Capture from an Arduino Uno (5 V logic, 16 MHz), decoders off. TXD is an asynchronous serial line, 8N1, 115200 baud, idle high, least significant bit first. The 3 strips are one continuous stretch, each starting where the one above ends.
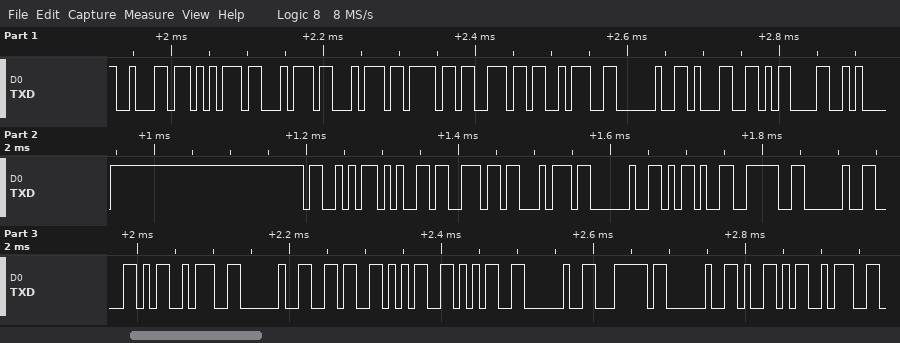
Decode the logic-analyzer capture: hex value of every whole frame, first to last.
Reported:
0x62 0x75 0x74 0x74 0x6F 0x6E 0x3A 0x20 0x31 0x0D 0x0A 0x53 0x65 0x6E 0x74 0x20 0x2D 0x3E 0x20 0x58 0x3A 0x20 0x36 0x35 0x35 0x20 0x7C 0x20 0x59 0x3A
